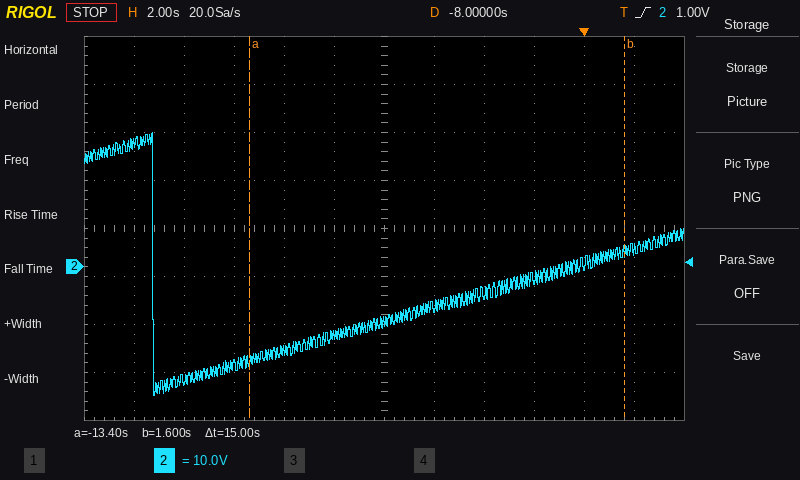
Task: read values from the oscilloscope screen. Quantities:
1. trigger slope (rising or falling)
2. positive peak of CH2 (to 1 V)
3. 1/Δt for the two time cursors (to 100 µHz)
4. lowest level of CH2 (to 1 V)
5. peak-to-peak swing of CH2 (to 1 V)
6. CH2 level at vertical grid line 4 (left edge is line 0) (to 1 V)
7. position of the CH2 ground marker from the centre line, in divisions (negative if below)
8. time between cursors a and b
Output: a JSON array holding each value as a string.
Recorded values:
["rising", "28 V", "66.7 mHz", "-27 V", "55 V", "-17 V", "-0.8 div", "15 s"]
